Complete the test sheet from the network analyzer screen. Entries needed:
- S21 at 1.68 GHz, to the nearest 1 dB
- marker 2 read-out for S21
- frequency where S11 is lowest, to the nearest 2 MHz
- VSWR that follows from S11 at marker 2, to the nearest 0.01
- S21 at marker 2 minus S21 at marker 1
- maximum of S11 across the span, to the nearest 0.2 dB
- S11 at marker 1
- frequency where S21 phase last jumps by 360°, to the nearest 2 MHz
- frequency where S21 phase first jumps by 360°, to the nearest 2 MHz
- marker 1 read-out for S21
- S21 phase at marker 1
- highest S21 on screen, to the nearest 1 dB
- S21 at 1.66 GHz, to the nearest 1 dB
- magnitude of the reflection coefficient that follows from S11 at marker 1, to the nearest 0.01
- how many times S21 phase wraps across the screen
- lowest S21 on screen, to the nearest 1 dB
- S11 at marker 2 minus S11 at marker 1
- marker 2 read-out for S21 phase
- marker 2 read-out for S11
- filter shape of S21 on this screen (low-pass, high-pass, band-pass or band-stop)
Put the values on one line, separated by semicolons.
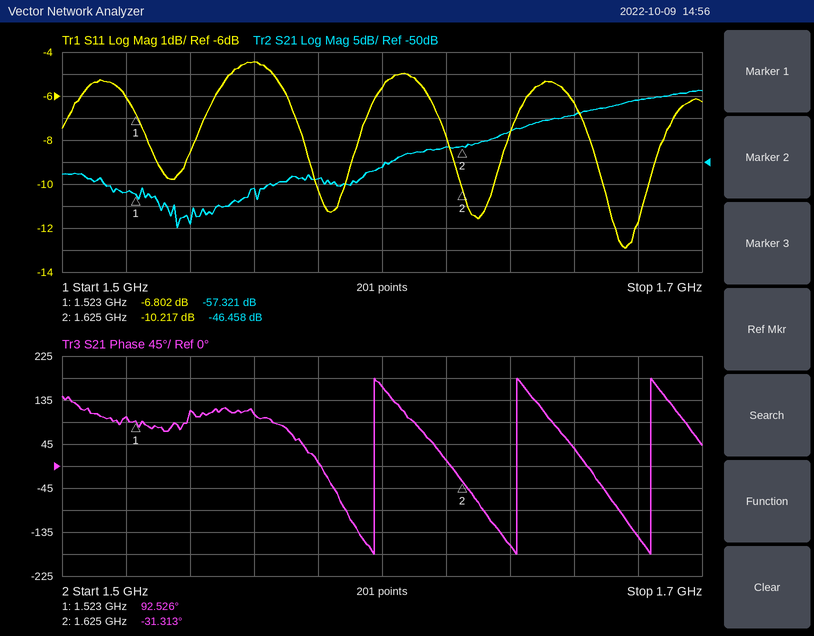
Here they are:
-36 dB; -46.458 dB; 1.676 GHz; 1.89; 10.863 dB; -4.4 dB; -6.802 dB; 1.684 GHz; 1.598 GHz; -57.321 dB; 92.526°; -34 dB; -39 dB; 0.46; 3; -65 dB; -3.415 dB; -31.313°; -10.217 dB; high-pass
